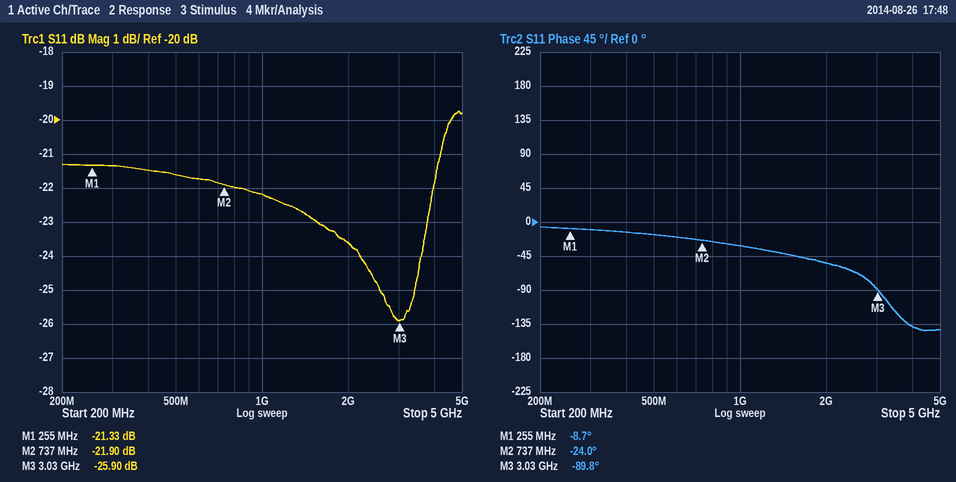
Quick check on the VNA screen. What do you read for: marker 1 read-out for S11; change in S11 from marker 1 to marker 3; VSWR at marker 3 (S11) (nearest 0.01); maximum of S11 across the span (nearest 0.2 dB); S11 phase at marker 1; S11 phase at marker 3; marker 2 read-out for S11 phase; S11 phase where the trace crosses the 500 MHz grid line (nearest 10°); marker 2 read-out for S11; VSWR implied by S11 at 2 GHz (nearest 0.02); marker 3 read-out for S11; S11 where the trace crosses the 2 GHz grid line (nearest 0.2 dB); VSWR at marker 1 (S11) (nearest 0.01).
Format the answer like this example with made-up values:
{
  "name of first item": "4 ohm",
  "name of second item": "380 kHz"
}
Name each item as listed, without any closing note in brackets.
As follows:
{
  "marker 1 read-out for S11": "-21.33 dB",
  "change in S11 from marker 1 to marker 3": "-4.57 dB",
  "VSWR at marker 3 (S11)": "1.11",
  "maximum of S11 across the span": "-19.8 dB",
  "S11 phase at marker 1": "-8.7°",
  "S11 phase at marker 3": "-89.8°",
  "marker 2 read-out for S11 phase": "-24.0°",
  "S11 phase where the trace crosses the 500 MHz grid line": "-20°",
  "marker 2 read-out for S11": "-21.90 dB",
  "VSWR implied by S11 at 2 GHz": "1.14",
  "marker 3 read-out for S11": "-25.90 dB",
  "S11 where the trace crosses the 2 GHz grid line": "-23.6 dB",
  "VSWR at marker 1 (S11)": "1.19"
}
